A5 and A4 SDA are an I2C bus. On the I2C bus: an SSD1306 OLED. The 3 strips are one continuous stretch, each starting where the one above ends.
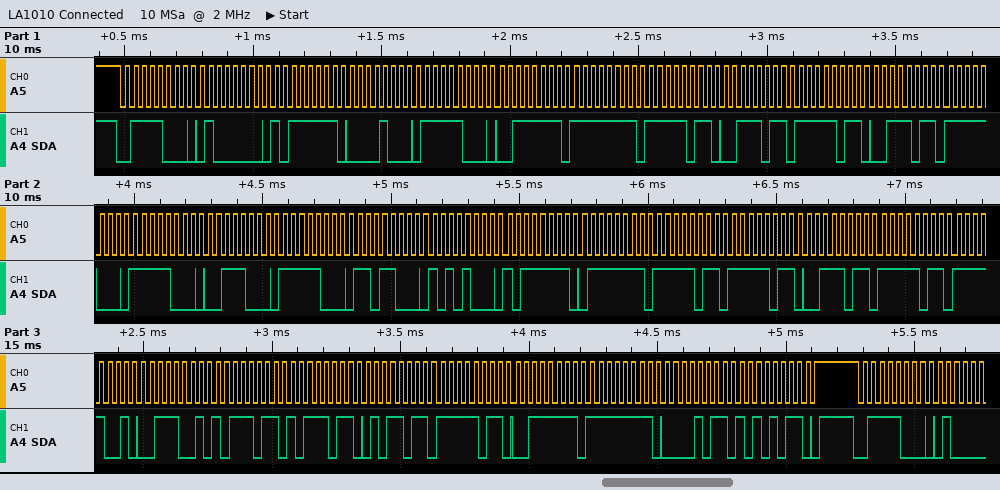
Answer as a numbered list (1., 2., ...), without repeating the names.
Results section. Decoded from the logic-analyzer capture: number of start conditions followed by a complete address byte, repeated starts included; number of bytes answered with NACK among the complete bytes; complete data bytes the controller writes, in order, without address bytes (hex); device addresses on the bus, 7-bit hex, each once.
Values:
1. 2
2. 0
3. 40 BF 08 F8 3F FF FB 3B FB 3B F8 F8 38 F8 D8 A8 BF 7F FB FB 3B FB F9 39 BB BB 5B FB 3F FF 0B AB
4. 0x3C
